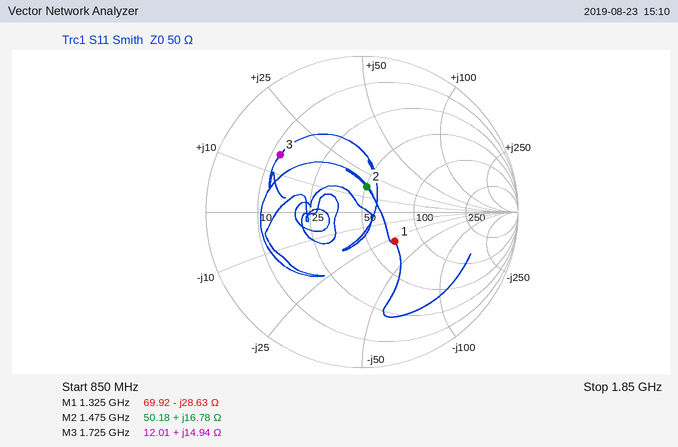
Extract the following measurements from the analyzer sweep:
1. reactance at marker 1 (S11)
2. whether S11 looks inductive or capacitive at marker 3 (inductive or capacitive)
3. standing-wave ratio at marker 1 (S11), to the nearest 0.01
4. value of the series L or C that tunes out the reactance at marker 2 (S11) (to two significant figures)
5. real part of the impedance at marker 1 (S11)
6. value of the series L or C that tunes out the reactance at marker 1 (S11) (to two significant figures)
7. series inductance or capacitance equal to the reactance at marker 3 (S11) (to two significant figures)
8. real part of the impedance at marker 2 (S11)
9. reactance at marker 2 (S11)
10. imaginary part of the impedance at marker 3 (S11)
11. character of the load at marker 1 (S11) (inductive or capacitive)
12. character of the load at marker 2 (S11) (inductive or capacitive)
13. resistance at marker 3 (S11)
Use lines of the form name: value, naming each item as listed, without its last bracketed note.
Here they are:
reactance at marker 1: -28.63 Ω
whether S11 looks inductive or capacitive at marker 3: inductive
standing-wave ratio at marker 1 (S11), to the nearest 0.01: 1.79
value of the series L or C that tunes out the reactance at marker 2 (S11): 6.4 pF
real part of the impedance at marker 1: 69.92 Ω
value of the series L or C that tunes out the reactance at marker 1 (S11): 3.4 nH
series inductance or capacitance equal to the reactance at marker 3 (S11): 1.4 nH
real part of the impedance at marker 2: 50.18 Ω
reactance at marker 2: +16.78 Ω
imaginary part of the impedance at marker 3: +14.94 Ω
character of the load at marker 1 (S11): capacitive
character of the load at marker 2 (S11): inductive
resistance at marker 3: 12.01 Ω
